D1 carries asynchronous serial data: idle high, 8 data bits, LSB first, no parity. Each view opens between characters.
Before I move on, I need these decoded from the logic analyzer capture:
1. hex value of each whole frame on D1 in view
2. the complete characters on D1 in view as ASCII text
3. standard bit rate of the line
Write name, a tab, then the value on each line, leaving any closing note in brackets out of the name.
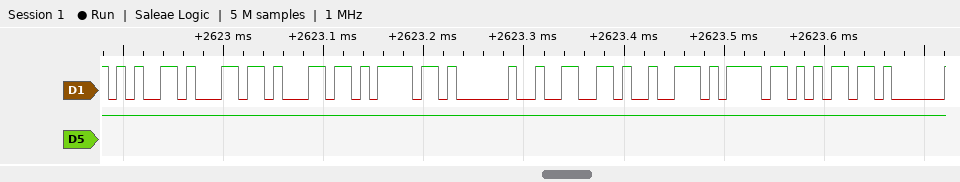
hex value of each whole frame on D1 in view	65, 6C, 6C, 6F, 20, 66, 72, 6F, 6D
the complete characters on D1 in view as ASCII text	"ello from"
standard bit rate of the line	115200 baud
